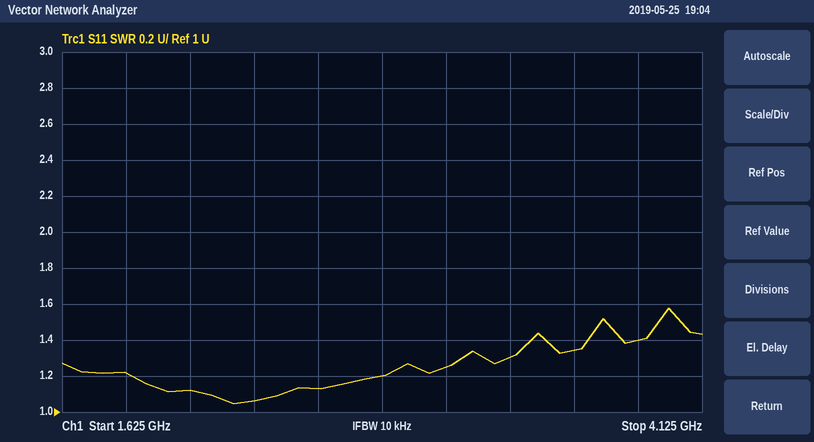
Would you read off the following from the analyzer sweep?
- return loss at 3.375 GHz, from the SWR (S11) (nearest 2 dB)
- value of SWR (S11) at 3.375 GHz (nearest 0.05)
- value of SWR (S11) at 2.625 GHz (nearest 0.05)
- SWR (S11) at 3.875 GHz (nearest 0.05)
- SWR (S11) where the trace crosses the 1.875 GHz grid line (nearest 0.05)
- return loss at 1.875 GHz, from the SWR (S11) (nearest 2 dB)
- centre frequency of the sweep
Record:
18 dB
1.30
1.15
1.40
1.20
20 dB
2.875 GHz
